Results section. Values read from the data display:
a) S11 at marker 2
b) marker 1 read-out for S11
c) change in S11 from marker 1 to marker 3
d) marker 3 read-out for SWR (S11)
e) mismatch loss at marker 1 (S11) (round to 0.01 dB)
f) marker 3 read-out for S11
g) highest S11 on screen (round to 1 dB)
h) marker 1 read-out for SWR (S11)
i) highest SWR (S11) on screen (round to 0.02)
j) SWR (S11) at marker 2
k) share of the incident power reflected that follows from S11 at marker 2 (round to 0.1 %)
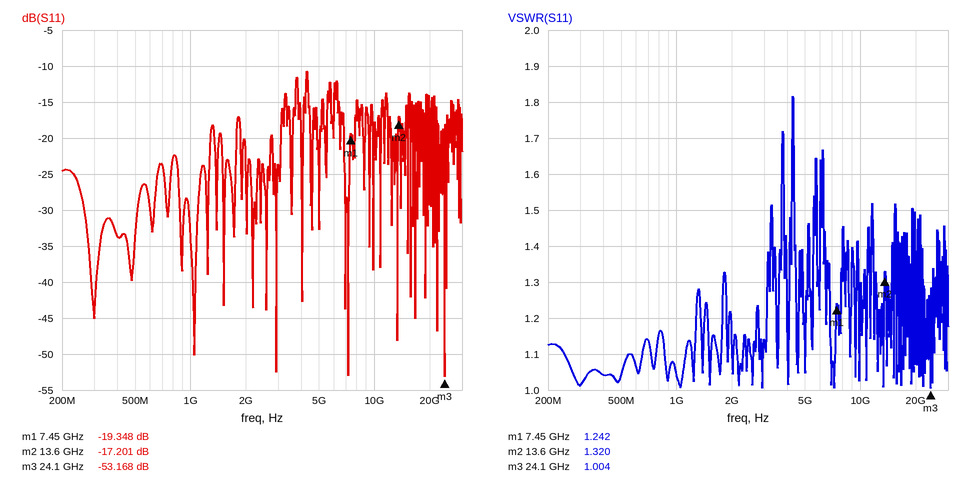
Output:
-17.201 dB
-19.348 dB
-33.820 dB
1.004
0.05 dB
-53.168 dB
-11 dB
1.242
1.82
1.320
1.9 %
